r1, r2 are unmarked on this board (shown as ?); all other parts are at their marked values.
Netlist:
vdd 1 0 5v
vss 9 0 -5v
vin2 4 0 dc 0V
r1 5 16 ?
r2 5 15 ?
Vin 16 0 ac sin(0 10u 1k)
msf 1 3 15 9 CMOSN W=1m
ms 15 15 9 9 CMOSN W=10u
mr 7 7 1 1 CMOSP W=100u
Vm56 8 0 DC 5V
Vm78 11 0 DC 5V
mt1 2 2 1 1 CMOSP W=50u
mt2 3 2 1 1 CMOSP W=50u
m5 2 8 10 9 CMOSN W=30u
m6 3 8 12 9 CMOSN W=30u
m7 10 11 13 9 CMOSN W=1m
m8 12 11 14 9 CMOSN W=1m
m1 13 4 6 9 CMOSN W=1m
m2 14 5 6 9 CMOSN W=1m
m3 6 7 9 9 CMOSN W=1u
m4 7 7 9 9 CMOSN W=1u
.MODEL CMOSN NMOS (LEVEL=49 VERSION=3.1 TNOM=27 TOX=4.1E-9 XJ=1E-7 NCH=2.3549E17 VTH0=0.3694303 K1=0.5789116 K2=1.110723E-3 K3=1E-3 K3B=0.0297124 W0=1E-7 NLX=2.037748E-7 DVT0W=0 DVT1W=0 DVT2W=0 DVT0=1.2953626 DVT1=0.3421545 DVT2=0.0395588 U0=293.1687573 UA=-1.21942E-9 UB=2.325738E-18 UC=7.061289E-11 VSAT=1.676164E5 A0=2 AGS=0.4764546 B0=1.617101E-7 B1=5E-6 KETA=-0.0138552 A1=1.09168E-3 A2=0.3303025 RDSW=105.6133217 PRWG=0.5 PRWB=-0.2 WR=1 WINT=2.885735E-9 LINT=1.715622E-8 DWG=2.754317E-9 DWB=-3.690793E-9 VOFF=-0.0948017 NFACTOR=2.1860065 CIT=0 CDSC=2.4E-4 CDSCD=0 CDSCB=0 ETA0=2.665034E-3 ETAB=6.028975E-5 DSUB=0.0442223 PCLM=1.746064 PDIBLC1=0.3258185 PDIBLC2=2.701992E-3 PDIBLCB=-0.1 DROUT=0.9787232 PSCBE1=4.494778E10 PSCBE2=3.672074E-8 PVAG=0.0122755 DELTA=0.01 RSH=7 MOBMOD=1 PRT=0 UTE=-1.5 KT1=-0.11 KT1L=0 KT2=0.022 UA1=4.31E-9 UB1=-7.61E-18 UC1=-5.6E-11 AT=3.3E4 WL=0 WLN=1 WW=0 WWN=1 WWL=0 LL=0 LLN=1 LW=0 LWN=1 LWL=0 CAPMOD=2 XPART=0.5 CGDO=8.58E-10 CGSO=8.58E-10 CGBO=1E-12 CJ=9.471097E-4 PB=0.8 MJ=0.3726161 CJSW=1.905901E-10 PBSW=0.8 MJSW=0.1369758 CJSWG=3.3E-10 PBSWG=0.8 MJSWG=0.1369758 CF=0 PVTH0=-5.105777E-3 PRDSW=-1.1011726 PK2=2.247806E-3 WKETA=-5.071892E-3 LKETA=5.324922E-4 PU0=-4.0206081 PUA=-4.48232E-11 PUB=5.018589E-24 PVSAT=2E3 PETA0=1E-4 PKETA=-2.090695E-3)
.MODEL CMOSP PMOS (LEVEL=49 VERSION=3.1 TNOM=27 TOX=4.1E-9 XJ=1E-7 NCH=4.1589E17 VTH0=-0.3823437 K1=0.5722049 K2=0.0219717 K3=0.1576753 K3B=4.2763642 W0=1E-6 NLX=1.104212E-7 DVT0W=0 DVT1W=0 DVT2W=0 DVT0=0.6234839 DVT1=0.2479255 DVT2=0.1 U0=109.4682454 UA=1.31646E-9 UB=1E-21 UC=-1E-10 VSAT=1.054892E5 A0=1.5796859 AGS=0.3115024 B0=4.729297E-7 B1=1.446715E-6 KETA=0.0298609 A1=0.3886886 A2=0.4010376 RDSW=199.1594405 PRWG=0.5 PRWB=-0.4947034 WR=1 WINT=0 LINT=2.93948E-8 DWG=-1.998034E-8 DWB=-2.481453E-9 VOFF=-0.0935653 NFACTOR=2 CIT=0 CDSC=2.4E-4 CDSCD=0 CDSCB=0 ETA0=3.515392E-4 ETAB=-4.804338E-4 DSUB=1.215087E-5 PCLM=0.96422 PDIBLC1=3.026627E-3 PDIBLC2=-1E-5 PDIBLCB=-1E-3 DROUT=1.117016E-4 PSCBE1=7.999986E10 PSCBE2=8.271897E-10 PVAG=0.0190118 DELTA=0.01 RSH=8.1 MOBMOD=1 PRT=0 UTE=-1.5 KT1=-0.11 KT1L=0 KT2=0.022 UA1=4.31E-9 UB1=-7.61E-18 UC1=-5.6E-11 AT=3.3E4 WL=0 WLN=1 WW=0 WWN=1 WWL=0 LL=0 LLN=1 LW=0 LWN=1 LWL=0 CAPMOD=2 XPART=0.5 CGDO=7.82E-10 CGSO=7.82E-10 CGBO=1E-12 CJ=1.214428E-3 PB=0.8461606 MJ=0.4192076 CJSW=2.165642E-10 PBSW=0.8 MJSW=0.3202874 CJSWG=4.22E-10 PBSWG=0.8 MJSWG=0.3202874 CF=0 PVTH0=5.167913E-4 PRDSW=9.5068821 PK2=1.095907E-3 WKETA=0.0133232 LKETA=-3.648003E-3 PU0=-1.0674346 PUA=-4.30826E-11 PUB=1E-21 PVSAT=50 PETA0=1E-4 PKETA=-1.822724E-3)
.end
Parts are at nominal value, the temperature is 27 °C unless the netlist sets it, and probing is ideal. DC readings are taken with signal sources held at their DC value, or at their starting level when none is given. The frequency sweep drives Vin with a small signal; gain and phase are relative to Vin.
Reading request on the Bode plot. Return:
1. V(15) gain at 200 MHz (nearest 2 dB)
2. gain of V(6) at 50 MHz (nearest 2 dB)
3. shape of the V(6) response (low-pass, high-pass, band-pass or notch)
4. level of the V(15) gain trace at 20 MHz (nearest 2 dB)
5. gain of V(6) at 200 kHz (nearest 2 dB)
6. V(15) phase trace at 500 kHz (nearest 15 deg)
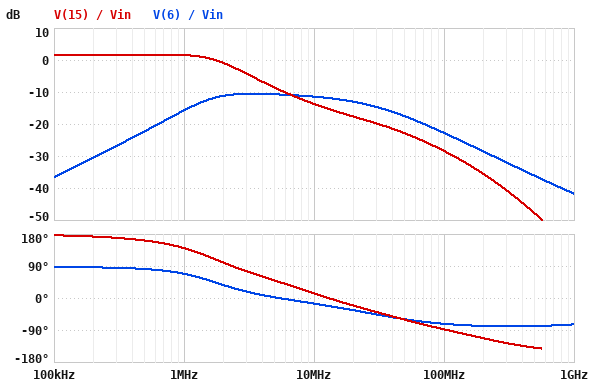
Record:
-36 dB
-18 dB
band-pass
-18 dB
-30 dB
165 deg
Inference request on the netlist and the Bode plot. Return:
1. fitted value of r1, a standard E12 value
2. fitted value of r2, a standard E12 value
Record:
680 Ω
820 Ω
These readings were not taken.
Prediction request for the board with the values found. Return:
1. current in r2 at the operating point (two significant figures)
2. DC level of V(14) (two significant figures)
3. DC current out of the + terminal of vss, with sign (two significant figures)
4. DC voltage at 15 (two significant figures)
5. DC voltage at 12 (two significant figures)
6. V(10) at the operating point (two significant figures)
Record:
6.9 µA
1.5 V
-3.0 mA
10 mV
1.5 V
3.1 V
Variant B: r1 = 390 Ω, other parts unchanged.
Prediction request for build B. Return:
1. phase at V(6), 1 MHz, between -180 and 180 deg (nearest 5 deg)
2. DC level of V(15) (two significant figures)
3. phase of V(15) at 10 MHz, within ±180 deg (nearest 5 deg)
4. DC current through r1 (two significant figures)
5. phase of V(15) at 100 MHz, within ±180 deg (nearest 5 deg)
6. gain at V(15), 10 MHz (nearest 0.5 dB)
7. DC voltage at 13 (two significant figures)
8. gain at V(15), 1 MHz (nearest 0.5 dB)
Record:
55 deg
15 mV
20 deg
12 µA
-80 deg
-12.0 dB
3.1 V
5.5 dB
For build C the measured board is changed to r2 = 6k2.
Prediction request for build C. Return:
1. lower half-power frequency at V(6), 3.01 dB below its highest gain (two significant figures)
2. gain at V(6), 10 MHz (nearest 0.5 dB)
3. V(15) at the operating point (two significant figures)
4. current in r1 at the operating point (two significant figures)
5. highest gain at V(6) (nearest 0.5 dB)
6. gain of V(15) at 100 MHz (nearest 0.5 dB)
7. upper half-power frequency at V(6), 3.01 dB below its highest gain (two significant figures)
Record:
380 kHz
-9.0 dB
47 mV
6.8 µA
-7.5 dB
-41.5 dB
17 MHz
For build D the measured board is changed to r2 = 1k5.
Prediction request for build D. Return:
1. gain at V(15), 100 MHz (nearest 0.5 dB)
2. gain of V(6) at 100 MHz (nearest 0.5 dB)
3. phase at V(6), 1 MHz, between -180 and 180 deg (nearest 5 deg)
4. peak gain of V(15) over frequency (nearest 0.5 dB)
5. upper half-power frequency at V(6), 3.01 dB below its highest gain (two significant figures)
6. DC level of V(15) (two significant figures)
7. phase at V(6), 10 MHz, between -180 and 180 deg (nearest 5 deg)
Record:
-32.5 dB
-22.5 dB
55 deg
7.0 dB
19 MHz
15 mV
-20 deg
